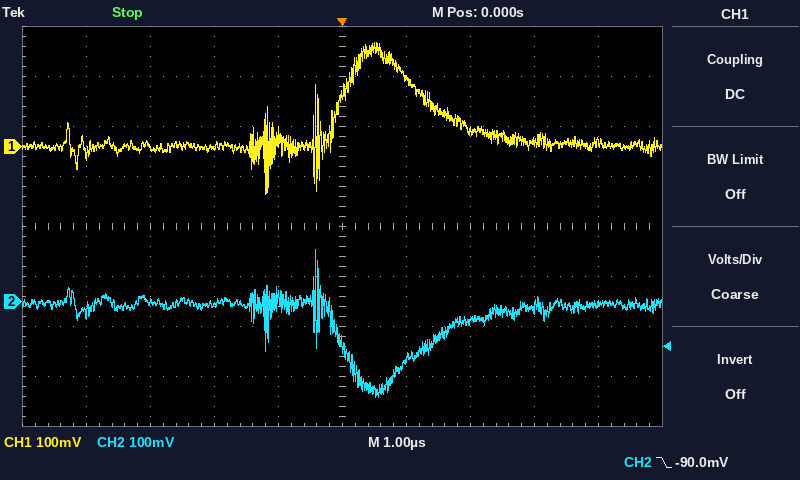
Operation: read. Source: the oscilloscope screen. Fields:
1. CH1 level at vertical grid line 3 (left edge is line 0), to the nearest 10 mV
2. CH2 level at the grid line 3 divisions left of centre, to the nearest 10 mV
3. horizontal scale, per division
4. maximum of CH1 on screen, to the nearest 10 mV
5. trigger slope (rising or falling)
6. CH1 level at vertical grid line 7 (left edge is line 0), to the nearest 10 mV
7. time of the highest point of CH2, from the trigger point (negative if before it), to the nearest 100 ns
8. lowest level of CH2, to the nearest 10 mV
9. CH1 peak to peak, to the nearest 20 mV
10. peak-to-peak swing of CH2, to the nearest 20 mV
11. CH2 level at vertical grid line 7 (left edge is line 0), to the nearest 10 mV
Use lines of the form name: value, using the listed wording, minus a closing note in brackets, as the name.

CH1 level at vertical grid line 3 (left edge is line 0), to the nearest 10 mV: 0 mV
CH2 level at the grid line 3 divisions left of centre, to the nearest 10 mV: 0 mV
horizontal scale, per division: 1 µs
maximum of CH1 on screen, to the nearest 10 mV: 210 mV
trigger slope: falling
CH1 level at vertical grid line 7 (left edge is line 0), to the nearest 10 mV: 30 mV
time of the highest point of CH2, from the trigger point (negative if before it), to the nearest 100 ns: -400 ns
lowest level of CH2, to the nearest 10 mV: -190 mV
CH1 peak to peak, to the nearest 20 mV: 300 mV
peak-to-peak swing of CH2, to the nearest 20 mV: 300 mV
CH2 level at vertical grid line 7 (left edge is line 0), to the nearest 10 mV: -40 mV
